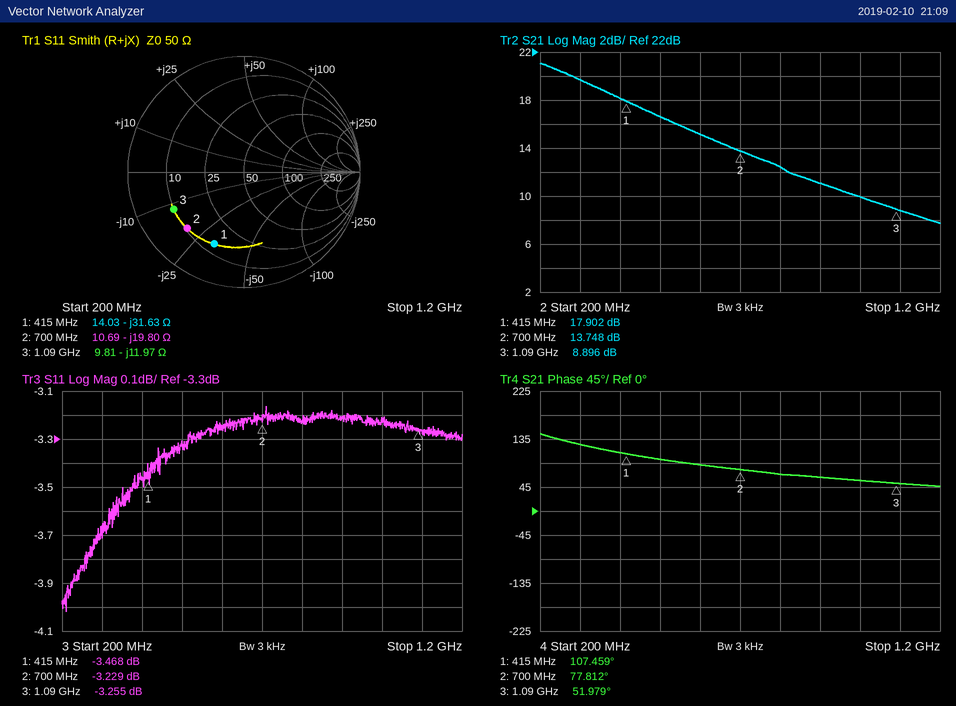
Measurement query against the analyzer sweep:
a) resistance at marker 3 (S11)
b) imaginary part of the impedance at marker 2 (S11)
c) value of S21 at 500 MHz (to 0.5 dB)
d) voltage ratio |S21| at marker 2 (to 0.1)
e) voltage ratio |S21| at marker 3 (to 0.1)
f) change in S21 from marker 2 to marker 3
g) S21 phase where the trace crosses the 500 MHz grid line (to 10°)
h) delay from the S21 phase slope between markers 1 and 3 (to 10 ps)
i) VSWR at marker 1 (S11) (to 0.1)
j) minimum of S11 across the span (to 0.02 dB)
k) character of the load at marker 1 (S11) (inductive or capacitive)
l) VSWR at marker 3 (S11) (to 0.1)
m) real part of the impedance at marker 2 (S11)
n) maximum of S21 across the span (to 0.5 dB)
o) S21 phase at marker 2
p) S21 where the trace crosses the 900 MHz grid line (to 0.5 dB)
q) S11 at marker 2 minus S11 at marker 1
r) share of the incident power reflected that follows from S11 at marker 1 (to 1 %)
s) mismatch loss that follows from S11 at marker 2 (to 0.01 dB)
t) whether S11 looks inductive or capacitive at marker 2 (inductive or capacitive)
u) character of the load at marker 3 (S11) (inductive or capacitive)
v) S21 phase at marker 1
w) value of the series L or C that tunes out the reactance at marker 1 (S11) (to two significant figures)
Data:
9.81 Ω
-19.80 Ω
16.5 dB
4.9
2.8
-4.852 dB
100°
230 ps
5.1
-4.02 dB
capacitive
5.4
10.69 Ω
21.0 dB
77.812°
11.0 dB
0.239 dB
45 %
2.80 dB
capacitive
capacitive
107.459°
12 nH
